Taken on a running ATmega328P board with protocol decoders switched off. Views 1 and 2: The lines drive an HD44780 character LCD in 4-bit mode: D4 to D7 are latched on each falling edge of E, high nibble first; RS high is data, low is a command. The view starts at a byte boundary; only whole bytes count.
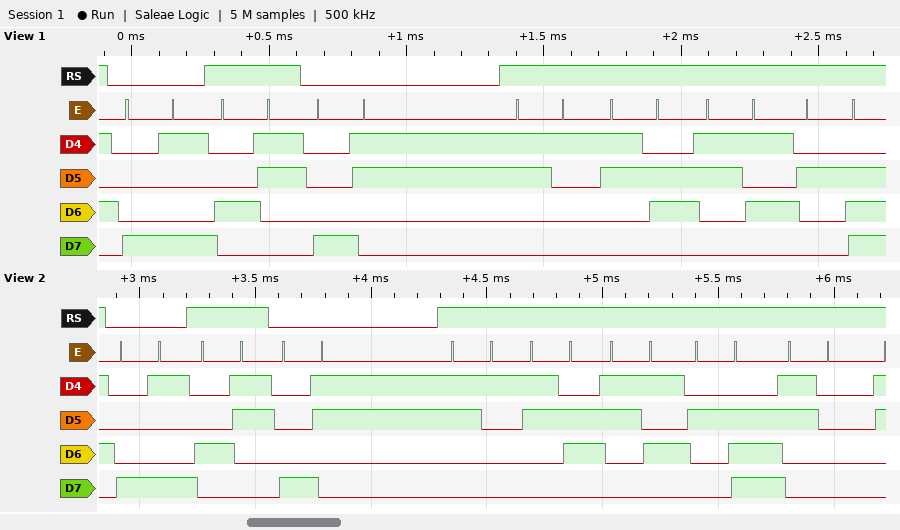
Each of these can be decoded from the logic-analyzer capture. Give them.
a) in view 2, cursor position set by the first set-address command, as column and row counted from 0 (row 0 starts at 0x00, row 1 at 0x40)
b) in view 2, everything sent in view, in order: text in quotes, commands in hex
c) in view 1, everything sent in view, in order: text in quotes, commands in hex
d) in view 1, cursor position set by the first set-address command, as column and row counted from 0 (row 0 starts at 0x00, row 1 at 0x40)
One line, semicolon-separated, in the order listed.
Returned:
column 9, row 0; 0x89 "C" 0x83 "165.0"; 0x89 "C" 0x83 "165."; column 9, row 0
